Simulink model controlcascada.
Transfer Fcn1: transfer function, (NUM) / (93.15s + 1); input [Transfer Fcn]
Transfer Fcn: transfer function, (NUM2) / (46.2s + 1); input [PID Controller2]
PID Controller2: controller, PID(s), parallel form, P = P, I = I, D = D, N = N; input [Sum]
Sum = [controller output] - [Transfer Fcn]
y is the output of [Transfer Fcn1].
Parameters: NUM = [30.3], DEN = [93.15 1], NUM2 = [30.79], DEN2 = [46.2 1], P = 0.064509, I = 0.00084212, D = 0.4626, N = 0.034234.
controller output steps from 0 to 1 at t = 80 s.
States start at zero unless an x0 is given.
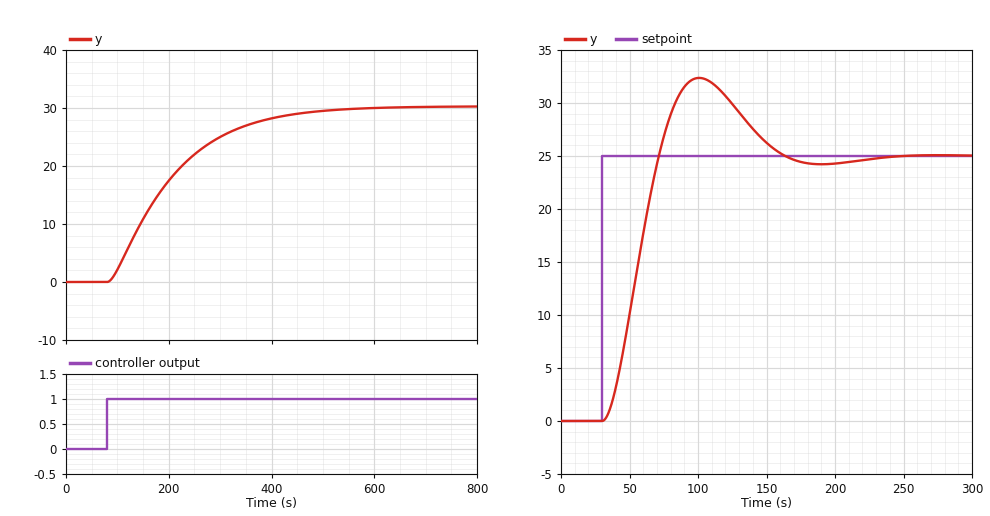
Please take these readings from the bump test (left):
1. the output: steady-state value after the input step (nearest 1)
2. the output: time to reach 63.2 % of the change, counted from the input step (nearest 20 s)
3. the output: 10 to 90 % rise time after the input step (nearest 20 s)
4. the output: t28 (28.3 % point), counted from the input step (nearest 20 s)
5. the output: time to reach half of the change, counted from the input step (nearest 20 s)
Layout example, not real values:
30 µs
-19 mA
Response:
30
140 s
260 s
60 s
100 s
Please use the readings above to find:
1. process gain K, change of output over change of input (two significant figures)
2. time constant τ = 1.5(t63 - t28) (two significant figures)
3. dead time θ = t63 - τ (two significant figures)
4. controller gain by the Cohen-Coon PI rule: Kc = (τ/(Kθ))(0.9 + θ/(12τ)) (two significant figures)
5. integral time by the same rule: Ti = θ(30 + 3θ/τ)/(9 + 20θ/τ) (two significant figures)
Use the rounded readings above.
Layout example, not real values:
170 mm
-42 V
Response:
30
120 s
20 s
0.18
49 s
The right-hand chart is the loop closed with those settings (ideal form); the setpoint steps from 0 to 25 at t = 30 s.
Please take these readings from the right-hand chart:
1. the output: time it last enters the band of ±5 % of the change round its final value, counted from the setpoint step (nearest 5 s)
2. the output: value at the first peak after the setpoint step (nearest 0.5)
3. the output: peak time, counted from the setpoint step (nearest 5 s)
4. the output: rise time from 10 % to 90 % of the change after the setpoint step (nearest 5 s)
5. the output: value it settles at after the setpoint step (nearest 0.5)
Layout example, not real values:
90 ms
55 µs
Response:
120 s
32.5
70 s
30 s
25.0
